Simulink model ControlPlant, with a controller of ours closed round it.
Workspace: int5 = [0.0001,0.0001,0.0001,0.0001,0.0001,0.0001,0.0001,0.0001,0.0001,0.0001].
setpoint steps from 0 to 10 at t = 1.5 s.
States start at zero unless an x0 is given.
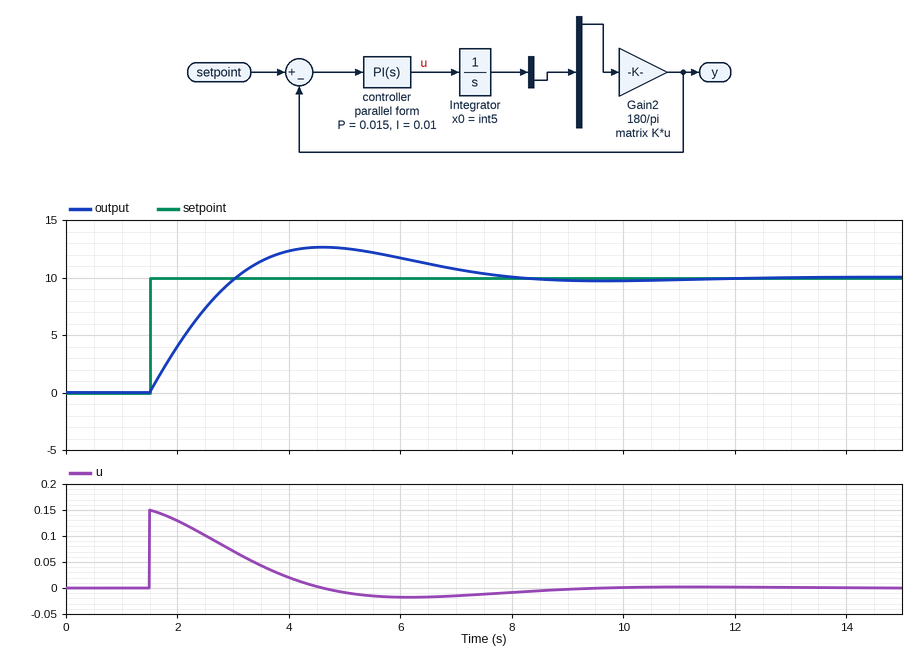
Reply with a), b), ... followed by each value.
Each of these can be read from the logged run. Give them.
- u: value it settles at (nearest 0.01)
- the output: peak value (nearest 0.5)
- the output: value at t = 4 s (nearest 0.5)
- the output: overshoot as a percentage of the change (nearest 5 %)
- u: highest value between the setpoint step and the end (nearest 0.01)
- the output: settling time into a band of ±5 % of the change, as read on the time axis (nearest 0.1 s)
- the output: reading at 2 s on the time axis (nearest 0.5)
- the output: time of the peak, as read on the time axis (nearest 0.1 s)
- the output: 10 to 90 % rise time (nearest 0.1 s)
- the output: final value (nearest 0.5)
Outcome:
a) 0.00
b) 12.5
c) 12.5
d) 25 %
e) 0.15
f) 7.3 s
g) 4.0
h) 4.6 s
i) 1.2 s
j) 10.0
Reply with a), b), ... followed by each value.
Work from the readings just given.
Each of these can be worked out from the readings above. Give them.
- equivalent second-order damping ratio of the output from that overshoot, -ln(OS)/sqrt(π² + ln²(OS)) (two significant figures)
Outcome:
a) 0.40
